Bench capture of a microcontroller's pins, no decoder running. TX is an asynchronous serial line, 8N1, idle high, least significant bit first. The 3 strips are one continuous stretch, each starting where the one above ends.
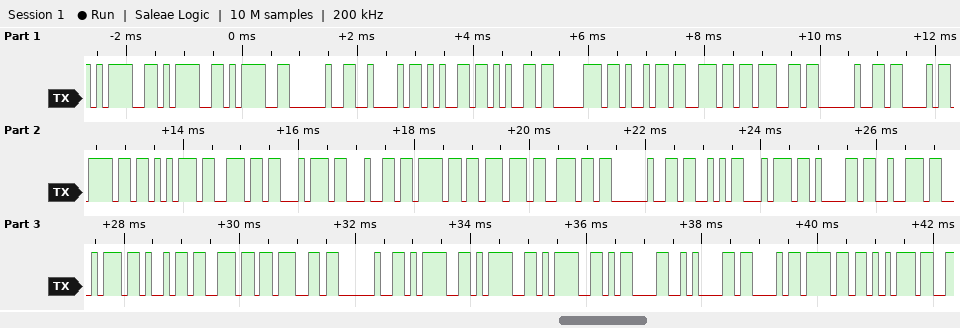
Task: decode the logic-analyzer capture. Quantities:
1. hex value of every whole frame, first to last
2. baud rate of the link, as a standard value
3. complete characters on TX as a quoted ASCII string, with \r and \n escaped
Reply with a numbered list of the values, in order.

1. 3D 3D 3D 20 42 65 65 70 69 6E 67 20 43 6F 75 6E 74 64 6F 77 6E 20 53 74 61 72 74 69 6E 67 20 3D 3D 3D 0D 0A 43 6F 75
2. 9600 baud
3. "=== Beeping Countdown Starting ===\r\nCou"
